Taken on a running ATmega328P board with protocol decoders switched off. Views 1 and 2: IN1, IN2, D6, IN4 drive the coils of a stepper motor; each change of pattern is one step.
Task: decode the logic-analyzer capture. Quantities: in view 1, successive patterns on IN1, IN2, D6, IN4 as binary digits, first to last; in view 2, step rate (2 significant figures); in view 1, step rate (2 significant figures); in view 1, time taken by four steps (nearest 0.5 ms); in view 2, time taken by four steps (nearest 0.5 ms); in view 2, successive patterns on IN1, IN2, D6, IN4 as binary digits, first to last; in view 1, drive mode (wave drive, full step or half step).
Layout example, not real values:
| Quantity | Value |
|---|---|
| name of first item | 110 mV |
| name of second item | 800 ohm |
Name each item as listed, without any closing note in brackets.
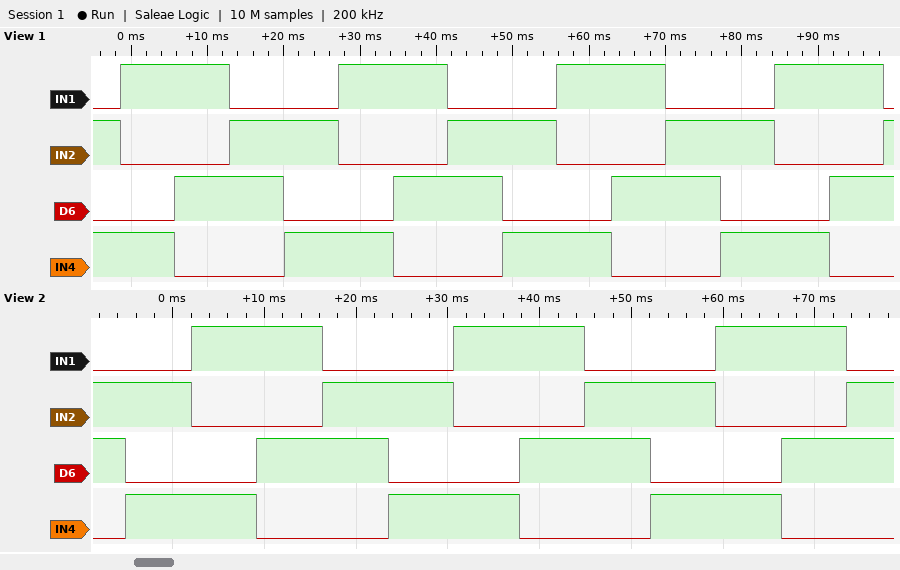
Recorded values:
| Quantity | Value |
|---|---|
| in view 1, successive patterns on IN1, IN2, D6, IN4 as binary digits, first to last | 0101 1001 1010 0110 0101 1001 1010 0110 0101 1001 1010 0110 0101 1001 1010 0110 |
| in view 2, step rate | 140 steps/s |
| in view 1, step rate | 140 steps/s |
| in view 1, time taken by four steps | 28.5 ms |
| in view 2, time taken by four steps | 28.5 ms |
| in view 2, successive patterns on IN1, IN2, D6, IN4 as binary digits, first to last | 0110 0101 1001 1010 0110 0101 1001 1010 0110 0101 1001 1010 0110 |
| in view 1, drive mode | full step |
